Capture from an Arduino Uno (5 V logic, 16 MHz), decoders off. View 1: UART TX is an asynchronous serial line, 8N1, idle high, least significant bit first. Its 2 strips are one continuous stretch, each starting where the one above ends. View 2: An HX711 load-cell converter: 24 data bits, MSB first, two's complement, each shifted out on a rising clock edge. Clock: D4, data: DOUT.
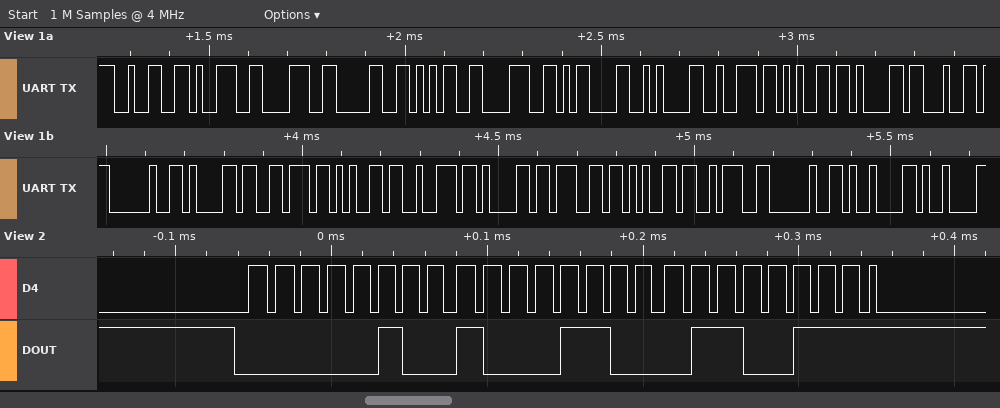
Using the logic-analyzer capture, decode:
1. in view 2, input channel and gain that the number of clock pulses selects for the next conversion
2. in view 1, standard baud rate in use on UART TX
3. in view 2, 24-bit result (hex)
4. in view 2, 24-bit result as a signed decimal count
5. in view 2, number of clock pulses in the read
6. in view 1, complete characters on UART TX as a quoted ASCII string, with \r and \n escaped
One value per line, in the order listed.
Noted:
channel A, gain 128
57600 baud
0x048C67
298087
25
"298058\r\nread average: \t\t"
